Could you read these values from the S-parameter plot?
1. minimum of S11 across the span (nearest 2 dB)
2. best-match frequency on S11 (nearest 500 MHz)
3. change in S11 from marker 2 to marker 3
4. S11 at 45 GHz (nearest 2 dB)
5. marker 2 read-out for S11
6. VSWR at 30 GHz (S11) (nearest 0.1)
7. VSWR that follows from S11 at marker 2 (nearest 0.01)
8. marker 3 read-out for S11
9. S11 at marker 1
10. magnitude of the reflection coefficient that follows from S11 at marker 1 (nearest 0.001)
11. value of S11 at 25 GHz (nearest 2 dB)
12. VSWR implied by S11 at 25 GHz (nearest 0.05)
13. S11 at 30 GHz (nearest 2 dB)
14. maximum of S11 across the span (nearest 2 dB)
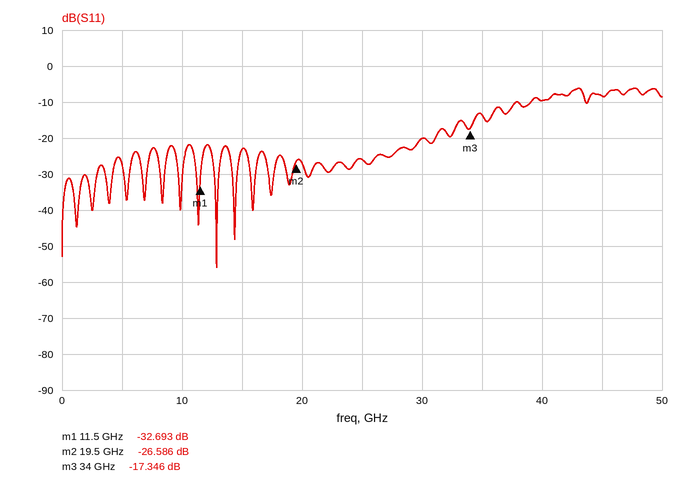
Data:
-56 dB
13.0 GHz
9.240 dB
-8 dB
-26.586 dB
1.2
1.10
-17.346 dB
-32.693 dB
0.023
-26 dB
1.10
-20 dB
-6 dB
